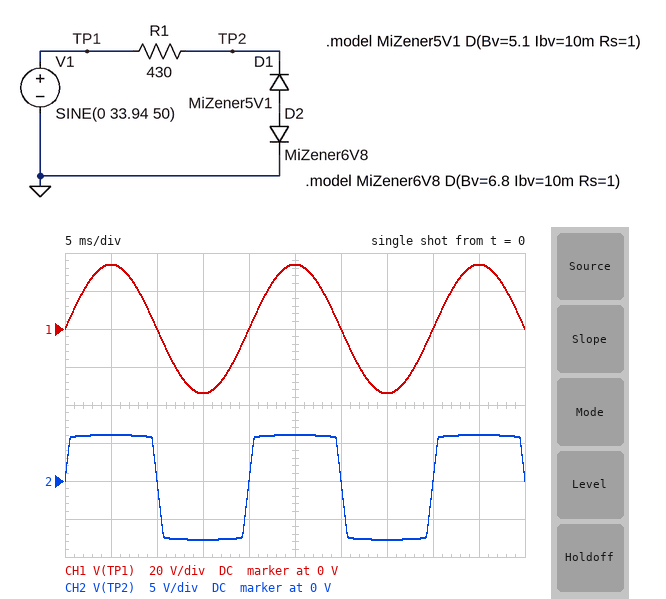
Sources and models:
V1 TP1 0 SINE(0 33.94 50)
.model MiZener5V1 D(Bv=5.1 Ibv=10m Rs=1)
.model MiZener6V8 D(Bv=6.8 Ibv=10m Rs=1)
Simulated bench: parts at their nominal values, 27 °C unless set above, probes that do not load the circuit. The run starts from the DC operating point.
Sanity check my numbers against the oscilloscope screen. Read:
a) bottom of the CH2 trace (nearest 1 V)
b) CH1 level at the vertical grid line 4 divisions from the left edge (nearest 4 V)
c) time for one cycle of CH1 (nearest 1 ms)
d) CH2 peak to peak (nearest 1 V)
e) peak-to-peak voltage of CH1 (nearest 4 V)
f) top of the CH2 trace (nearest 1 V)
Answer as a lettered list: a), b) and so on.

a) -8 V
b) 0 V
c) 20 ms
d) 14 V
e) 68 V
f) 6 V
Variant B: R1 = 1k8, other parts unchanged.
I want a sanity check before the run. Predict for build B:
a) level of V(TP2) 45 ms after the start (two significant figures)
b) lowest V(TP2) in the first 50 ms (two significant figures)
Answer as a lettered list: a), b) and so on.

a) 5.9 V
b) -7.6 V
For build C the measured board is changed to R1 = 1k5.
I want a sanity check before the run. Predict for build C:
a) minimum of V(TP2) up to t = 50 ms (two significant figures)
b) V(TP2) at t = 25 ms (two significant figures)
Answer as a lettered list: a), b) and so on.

a) -7.6 V
b) 5.9 V
